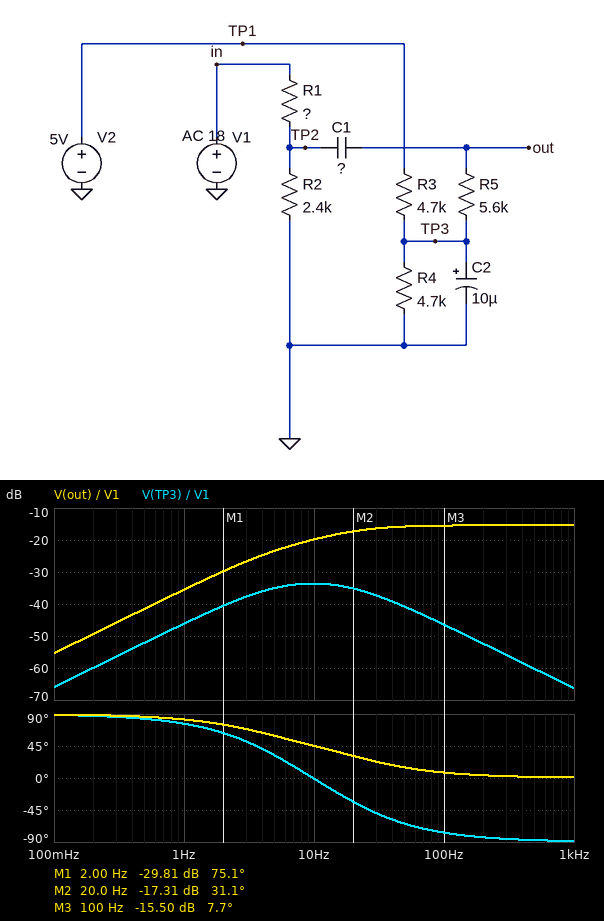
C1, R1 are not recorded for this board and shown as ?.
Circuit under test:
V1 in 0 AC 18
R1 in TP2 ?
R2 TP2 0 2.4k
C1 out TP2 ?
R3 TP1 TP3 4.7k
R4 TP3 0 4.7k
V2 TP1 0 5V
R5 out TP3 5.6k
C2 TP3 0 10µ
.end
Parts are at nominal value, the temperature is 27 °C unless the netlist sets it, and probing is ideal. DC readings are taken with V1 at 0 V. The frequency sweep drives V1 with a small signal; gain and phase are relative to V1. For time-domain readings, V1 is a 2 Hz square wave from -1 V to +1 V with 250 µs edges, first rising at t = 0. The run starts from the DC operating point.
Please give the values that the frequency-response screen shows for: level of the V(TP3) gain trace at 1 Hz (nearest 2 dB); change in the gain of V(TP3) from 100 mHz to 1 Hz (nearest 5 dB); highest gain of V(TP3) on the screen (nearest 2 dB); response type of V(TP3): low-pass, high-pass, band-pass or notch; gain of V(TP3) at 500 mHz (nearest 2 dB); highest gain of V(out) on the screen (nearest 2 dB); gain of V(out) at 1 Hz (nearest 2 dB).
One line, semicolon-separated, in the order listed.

-46 dB; 20 dB; -34 dB; band-pass; -52 dB; -16 dB; -36 dB
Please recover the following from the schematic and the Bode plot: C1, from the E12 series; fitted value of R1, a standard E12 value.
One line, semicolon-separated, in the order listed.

1.5 µF; 8.2 kΩ
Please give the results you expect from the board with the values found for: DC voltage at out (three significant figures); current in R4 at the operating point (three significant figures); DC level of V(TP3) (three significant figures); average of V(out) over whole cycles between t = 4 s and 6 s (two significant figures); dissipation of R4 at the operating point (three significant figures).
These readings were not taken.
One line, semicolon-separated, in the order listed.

2.50 V; 532 µA; 2.50 V; 2.5 V; 1.33 mW
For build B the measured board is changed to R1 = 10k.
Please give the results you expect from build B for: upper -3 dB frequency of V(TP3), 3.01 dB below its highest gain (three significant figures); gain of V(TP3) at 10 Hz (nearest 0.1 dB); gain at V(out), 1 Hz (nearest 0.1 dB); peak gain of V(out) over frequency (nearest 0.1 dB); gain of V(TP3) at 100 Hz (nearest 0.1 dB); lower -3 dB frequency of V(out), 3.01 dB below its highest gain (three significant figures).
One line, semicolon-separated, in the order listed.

26.6 Hz; -35.0 dB; -36.9 dB; -16.8 dB; -47.9 dB; 14.1 Hz
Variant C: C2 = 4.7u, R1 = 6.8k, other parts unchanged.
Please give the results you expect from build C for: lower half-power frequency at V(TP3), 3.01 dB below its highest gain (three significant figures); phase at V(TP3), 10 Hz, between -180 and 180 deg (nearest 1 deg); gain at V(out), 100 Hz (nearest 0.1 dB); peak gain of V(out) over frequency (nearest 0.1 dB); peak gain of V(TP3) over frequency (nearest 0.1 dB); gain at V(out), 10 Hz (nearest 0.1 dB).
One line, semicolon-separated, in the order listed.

5.35 Hz; 18 deg; -14.2 dB; -14.1 dB; -28.9 dB; -17.8 dB
